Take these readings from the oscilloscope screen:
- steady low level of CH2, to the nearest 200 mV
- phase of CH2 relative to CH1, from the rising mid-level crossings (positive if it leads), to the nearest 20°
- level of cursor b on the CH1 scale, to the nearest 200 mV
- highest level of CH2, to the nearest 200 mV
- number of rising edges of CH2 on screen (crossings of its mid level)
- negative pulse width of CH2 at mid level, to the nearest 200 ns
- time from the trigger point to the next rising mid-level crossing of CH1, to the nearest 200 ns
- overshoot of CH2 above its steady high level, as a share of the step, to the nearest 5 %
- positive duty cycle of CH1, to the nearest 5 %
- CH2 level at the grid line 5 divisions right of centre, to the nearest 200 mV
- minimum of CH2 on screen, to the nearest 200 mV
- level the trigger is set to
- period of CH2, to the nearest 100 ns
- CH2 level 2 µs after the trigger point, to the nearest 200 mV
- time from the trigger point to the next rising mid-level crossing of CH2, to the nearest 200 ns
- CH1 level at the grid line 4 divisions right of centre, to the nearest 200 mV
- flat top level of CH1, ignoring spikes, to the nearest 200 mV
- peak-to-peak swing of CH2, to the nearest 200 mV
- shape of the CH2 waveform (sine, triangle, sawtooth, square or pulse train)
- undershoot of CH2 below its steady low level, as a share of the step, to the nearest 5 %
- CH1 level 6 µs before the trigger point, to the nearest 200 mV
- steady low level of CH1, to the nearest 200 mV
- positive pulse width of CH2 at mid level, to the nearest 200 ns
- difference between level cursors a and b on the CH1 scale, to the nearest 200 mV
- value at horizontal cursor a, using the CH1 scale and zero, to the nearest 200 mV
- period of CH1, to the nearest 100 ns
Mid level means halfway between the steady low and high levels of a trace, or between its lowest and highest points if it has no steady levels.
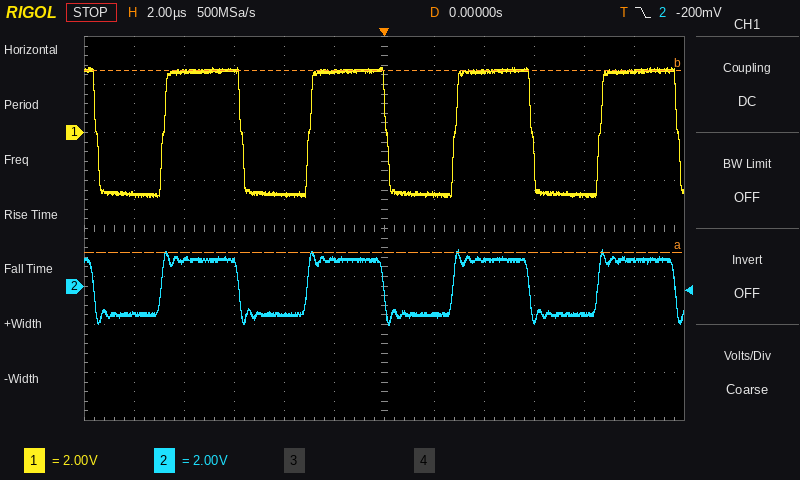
-1.2 V
0°
2.6 V
1.6 V
4
2.8 µs
2.8 µs
20 %
55 %
1.0 V
-1.6 V
-200 mV
5.8 µs
-1.2 V
2.8 µs
-2.6 V
2.6 V
3.2 V
square
20 %
2.6 V
-2.6 V
3.0 µs
7.6 V
-5.0 V
5.8 µs
